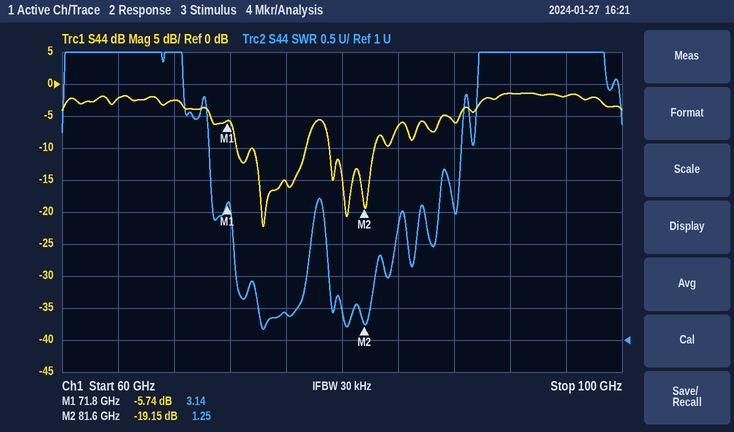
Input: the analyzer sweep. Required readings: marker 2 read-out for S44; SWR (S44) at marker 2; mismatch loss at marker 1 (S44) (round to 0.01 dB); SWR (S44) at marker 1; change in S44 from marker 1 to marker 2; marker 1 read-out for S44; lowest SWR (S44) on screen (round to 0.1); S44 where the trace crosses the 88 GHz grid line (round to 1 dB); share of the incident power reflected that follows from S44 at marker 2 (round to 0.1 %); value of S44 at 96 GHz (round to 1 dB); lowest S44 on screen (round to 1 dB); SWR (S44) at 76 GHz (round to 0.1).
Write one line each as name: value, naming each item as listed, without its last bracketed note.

marker 2 read-out for S44: -19.15 dB
SWR (S44) at marker 2: 1.25
mismatch loss at marker 1 (S44): 1.35 dB
SWR (S44) at marker 1: 3.14
change in S44 from marker 1 to marker 2: -13.41 dB
marker 1 read-out for S44: -5.74 dB
lowest SWR (S44) on screen: 1.2
S44 where the trace crosses the 88 GHz grid line: -6 dB
share of the incident power reflected that follows from S44 at marker 2: 1.2 %
value of S44 at 96 GHz: -2 dB
lowest S44 on screen: -22 dB
SWR (S44) at 76 GHz: 1.4
